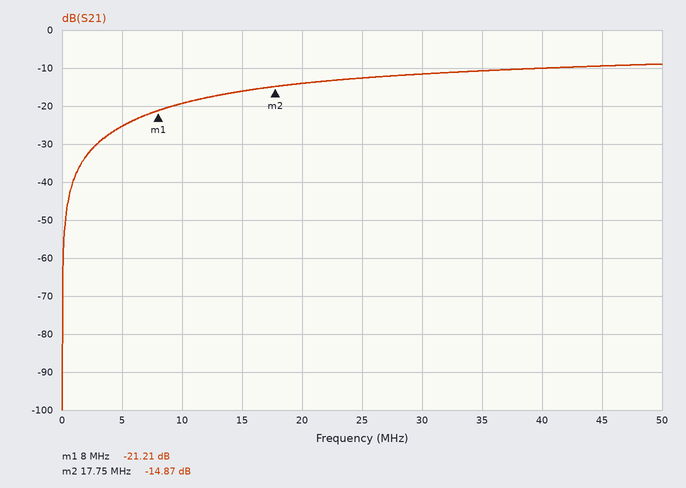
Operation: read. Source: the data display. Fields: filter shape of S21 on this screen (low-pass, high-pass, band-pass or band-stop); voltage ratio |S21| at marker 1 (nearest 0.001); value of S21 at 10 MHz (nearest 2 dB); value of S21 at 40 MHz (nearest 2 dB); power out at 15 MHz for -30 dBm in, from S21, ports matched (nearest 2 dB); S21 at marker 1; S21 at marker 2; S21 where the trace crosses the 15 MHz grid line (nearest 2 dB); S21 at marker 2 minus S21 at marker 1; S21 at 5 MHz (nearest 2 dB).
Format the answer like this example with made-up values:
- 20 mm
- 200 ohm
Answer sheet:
- high-pass
- 0.087
- -20 dB
- -10 dB
- -46 dBm
- -21.21 dB
- -14.87 dB
- -16 dB
- 6.34 dB
- -26 dB
